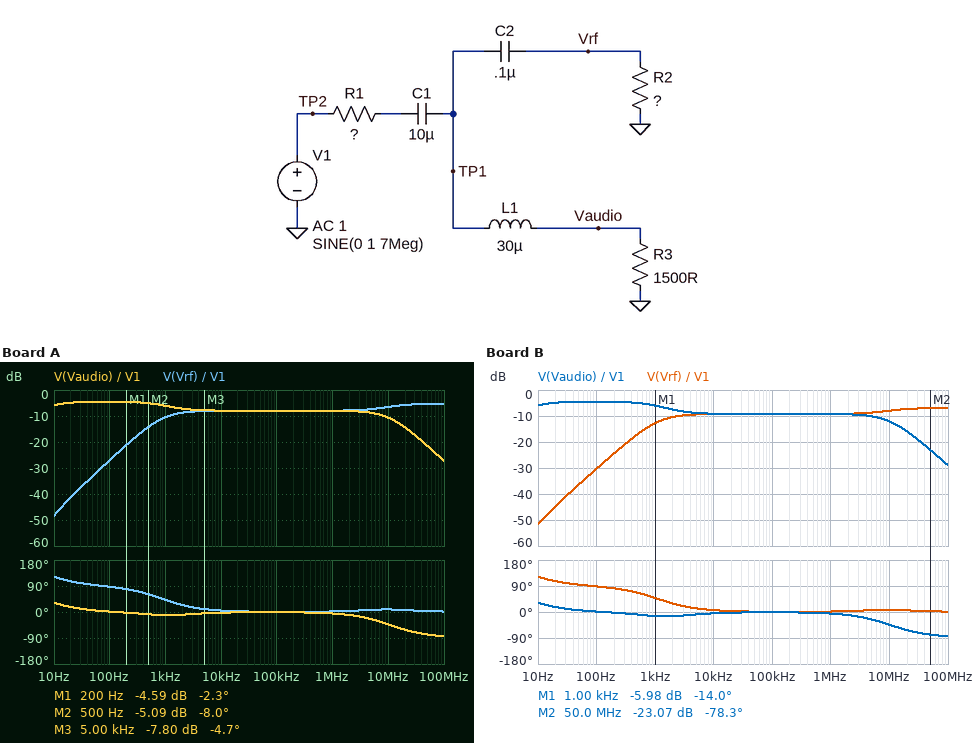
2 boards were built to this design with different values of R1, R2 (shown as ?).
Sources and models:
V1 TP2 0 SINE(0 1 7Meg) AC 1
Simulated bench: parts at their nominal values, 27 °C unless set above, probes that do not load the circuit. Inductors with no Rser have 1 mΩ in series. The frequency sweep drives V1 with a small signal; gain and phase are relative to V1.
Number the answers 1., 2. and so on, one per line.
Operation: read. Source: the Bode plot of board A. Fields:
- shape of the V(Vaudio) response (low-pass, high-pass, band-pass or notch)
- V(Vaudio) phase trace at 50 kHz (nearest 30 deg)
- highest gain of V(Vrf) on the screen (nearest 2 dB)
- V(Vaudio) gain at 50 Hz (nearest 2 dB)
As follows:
1. low-pass
2. 0 deg
3. -6 dB
4. -4 dB
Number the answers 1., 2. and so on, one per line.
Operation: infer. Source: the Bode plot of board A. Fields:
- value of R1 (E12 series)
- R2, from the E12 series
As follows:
1. 1 kΩ
2. 1.2 kΩ
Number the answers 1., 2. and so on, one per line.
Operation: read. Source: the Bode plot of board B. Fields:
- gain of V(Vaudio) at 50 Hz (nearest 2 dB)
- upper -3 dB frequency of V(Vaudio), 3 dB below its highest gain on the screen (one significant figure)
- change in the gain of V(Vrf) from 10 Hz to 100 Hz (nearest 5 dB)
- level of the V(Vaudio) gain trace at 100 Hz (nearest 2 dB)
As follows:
1. -4 dB
2. 2 kHz
3. 20 dB
4. -4 dB
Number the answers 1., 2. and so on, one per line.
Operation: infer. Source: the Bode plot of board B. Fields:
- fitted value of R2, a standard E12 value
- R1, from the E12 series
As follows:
1. 820 Ω
2. 1 kΩ
